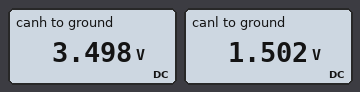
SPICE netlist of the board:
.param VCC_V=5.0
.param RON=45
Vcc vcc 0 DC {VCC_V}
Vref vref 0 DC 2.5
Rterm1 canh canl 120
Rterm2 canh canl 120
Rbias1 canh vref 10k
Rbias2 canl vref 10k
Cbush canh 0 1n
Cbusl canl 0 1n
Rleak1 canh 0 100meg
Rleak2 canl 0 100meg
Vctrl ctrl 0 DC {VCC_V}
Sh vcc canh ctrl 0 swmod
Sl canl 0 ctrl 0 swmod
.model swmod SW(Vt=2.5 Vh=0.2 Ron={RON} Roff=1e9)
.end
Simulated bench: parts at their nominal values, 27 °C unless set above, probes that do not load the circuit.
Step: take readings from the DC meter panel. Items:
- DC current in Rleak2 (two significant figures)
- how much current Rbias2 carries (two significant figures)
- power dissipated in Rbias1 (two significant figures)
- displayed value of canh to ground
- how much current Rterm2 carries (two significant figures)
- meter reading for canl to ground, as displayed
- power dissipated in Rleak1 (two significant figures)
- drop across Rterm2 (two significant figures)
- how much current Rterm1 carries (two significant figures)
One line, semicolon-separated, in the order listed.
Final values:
15 nA; 100 µA; 100 µW; 3.498 V; 17 mA; 1.502 V; 120 nW; 2.0 V; 17 mA
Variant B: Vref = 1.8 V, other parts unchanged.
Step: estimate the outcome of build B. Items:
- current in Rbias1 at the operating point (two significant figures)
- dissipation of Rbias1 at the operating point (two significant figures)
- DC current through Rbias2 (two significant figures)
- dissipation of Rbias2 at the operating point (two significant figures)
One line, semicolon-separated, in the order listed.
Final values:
170 µA; 290 µW; 30 µA; 9.1 µW
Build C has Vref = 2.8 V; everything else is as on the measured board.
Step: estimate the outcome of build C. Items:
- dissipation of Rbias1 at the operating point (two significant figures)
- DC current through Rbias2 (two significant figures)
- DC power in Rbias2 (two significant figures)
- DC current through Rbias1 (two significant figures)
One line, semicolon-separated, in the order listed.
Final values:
49 µW; 130 µA; 170 µW; 70 µA
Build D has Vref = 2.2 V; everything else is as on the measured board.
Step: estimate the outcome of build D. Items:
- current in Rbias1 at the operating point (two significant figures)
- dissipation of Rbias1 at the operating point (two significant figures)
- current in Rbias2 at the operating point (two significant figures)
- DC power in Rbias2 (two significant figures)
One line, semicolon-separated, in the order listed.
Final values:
130 µA; 170 µW; 70 µA; 49 µW
